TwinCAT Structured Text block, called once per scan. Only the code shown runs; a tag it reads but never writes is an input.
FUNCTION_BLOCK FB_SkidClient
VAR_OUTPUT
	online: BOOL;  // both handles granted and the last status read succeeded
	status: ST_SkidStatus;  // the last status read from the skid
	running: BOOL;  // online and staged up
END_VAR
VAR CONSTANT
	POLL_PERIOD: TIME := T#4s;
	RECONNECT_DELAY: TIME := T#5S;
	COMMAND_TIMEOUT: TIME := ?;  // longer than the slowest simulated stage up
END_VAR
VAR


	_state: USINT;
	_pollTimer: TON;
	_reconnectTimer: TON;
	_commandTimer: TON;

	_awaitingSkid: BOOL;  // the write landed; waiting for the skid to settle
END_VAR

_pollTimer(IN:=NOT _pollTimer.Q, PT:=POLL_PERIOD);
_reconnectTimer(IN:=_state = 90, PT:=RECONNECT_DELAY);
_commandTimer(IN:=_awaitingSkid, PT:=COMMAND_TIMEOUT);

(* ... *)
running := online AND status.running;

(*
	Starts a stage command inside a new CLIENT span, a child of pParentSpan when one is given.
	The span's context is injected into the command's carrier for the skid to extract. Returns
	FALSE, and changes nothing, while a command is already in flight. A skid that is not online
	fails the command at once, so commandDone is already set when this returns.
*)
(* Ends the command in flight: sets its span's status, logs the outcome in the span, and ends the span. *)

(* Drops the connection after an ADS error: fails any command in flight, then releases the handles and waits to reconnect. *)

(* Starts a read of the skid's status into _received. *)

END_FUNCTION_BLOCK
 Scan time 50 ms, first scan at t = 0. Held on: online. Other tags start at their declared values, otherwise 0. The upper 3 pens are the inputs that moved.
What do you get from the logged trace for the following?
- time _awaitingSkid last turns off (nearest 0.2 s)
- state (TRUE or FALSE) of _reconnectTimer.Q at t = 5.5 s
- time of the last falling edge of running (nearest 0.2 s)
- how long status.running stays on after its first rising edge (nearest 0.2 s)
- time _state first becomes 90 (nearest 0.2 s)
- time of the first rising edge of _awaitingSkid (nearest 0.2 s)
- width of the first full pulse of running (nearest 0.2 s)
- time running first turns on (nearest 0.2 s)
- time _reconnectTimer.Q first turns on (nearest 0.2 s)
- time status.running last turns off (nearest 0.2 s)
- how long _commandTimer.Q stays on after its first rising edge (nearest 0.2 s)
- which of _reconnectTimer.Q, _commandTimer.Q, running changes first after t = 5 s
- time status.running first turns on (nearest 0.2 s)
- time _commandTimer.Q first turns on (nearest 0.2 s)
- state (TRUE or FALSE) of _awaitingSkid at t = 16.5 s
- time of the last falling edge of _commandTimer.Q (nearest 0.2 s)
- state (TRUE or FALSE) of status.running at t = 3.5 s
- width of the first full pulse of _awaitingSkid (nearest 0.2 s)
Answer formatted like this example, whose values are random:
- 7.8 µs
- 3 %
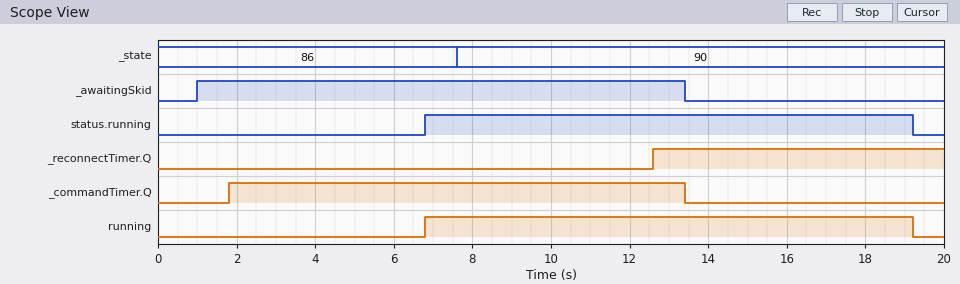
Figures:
- 13.4 s
- FALSE
- 19.2 s
- 12.4 s
- 7.6 s
- 1.0 s
- 12.4 s
- 6.8 s
- 12.6 s
- 19.2 s
- 11.6 s
- running
- 6.8 s
- 1.8 s
- FALSE
- 13.4 s
- FALSE
- 12.4 s
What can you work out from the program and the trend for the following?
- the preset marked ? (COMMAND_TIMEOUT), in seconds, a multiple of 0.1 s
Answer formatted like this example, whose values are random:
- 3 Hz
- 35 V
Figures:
- 0.8 s
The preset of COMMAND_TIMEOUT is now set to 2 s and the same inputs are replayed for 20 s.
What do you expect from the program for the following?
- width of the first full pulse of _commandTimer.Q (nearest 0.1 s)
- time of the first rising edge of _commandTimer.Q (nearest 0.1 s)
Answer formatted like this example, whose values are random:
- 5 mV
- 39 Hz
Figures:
- 10.4 s
- 3.0 s
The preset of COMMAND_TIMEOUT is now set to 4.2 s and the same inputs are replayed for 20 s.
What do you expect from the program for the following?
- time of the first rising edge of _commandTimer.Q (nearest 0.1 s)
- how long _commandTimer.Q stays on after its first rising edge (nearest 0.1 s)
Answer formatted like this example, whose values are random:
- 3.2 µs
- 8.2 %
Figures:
- 5.2 s
- 8.2 s
